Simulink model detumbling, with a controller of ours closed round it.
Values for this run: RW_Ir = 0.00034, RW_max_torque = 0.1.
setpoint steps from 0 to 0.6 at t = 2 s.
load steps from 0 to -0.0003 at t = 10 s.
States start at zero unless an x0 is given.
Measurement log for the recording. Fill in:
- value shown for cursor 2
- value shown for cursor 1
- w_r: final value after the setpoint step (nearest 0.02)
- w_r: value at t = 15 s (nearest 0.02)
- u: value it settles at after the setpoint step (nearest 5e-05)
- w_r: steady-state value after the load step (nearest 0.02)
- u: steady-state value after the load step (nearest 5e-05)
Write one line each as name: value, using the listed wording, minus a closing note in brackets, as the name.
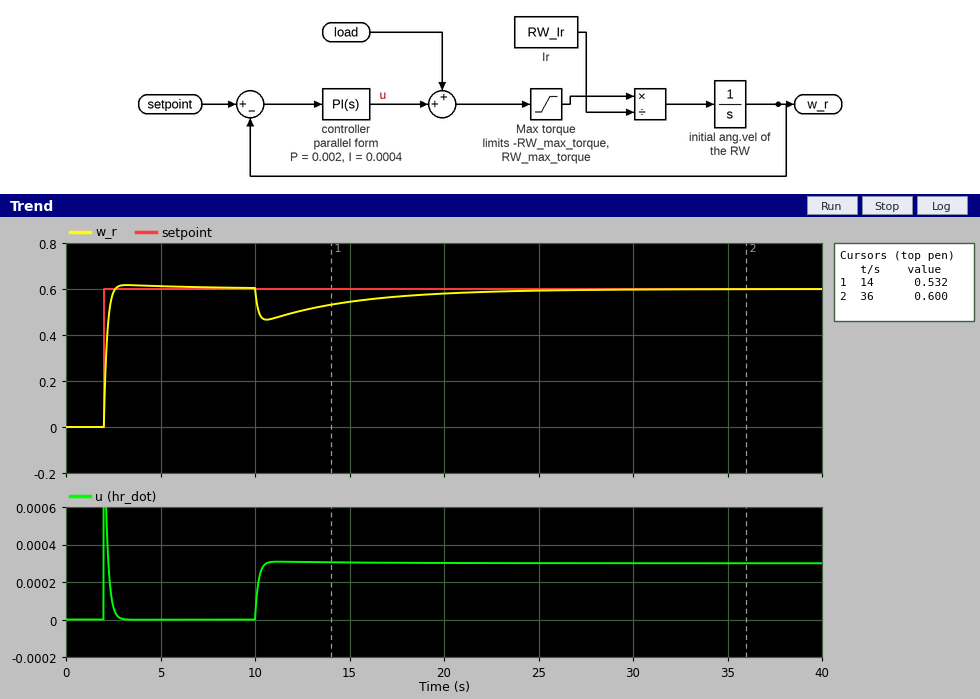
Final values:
value shown for cursor 2: 0.600
value shown for cursor 1: 0.532
w_r: final value after the setpoint step: 0.60
w_r: value at t = 15 s: 0.54
u: value it settles at after the setpoint step: 0.00000
w_r: steady-state value after the load step: 0.60
u: steady-state value after the load step: 0.00030
